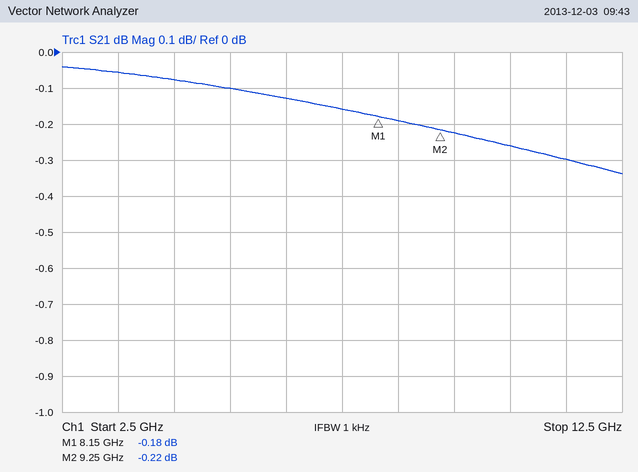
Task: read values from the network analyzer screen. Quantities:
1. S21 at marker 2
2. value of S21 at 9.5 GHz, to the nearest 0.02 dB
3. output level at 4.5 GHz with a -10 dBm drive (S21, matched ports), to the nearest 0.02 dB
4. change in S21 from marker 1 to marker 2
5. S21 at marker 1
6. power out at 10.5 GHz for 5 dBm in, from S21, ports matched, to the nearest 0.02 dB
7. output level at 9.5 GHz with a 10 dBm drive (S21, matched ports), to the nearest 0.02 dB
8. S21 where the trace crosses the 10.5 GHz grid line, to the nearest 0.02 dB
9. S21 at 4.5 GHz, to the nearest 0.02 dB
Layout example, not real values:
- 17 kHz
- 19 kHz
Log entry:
- -0.22 dB
- -0.22 dB
- -10.08 dBm
- -0.04 dB
- -0.18 dB
- 4.74 dBm
- 9.78 dBm
- -0.26 dB
- -0.08 dB
